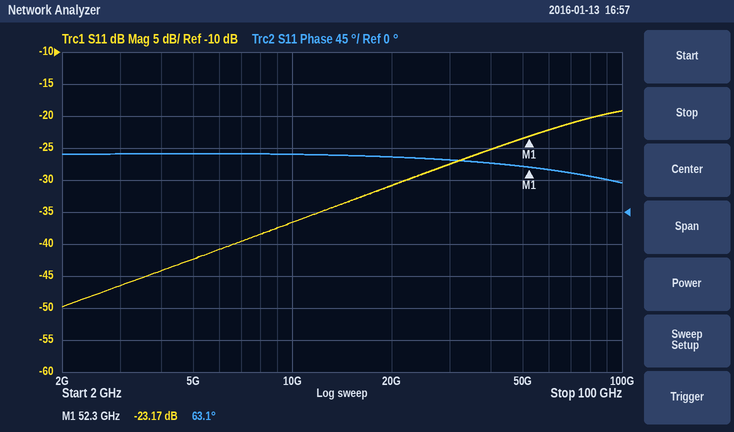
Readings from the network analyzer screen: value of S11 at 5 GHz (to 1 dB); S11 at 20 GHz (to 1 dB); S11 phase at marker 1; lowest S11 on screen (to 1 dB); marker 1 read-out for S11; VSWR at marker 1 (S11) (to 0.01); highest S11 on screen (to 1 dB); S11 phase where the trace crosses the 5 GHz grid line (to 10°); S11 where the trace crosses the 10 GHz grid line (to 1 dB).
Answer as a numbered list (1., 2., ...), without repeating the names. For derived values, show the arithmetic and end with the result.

1. -42 dB
2. -31 dB
3. 63.1°
4. -50 dB
5. -23.17 dB
6. (1 + 0.0694)/(1 − 0.0694) ≈ 1.15
7. -19 dB
8. 80°
9. -37 dB
